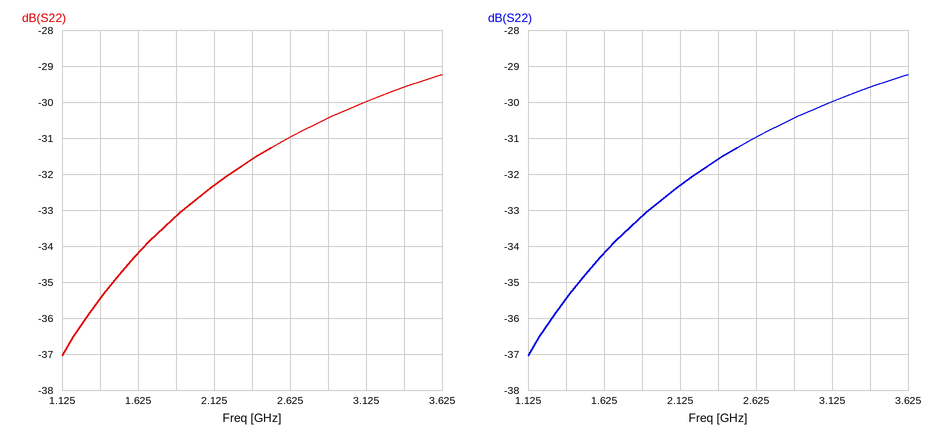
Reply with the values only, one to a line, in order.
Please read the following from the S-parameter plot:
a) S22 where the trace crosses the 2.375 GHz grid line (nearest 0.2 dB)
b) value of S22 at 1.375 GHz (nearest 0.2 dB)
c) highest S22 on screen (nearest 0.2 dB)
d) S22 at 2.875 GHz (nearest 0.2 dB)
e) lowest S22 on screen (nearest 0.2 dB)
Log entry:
-31.6 dB
-35.4 dB
-29.2 dB
-30.4 dB
-37.0 dB
